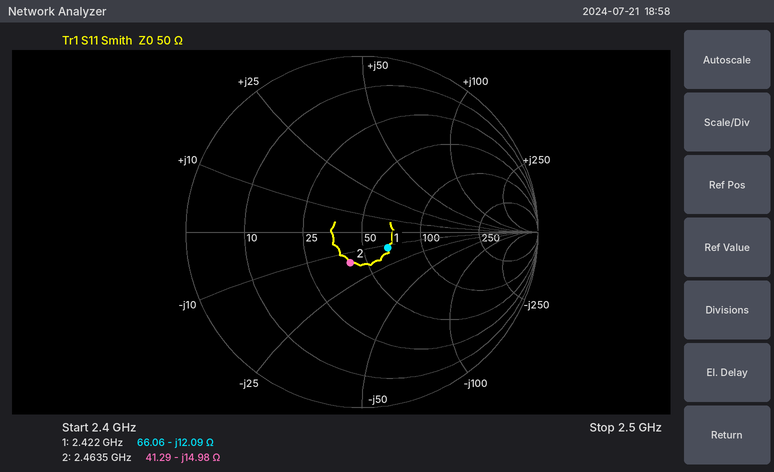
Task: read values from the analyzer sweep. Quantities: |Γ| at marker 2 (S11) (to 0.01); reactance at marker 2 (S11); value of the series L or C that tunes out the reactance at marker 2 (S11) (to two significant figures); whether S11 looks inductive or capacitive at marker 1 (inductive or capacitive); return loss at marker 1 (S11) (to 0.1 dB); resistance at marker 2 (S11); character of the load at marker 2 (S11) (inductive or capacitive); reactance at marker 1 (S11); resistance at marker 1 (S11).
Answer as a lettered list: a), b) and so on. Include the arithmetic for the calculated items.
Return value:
a) 0.19
b) -14.98 Ω
c) L = 14.98 Ω/(2π × 2.4635 GHz) ≈ 968 pH, so 970 pH to two significant figures
d) capacitive
e) 15.3 dB
f) 41.29 Ω
g) capacitive
h) -12.09 Ω
i) 66.06 Ω
